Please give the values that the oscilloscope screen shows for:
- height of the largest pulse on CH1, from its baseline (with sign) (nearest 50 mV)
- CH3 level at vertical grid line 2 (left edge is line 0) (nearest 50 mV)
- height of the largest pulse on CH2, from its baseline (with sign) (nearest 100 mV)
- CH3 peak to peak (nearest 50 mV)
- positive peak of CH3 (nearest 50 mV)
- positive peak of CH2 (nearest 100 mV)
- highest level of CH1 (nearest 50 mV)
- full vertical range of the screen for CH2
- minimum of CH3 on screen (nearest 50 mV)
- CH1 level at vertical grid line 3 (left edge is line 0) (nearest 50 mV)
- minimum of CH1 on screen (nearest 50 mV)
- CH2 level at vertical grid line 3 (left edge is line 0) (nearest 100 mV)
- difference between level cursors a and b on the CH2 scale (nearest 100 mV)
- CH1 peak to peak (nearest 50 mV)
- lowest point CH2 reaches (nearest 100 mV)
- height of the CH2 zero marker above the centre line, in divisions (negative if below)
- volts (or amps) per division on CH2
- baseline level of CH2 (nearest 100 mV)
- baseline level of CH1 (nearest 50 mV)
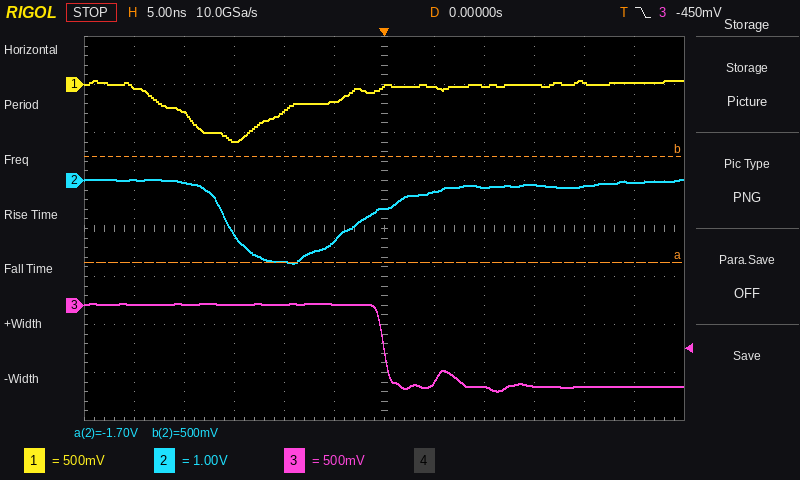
-600 mV
0 mV
-1.6 V
900 mV
0 mV
0.0 V
50 mV
8 V
-900 mV
-600 mV
-600 mV
-1.1 V
2.2 V
650 mV
-1.7 V
+1.0 div
1 V
-100 mV
0 mV
